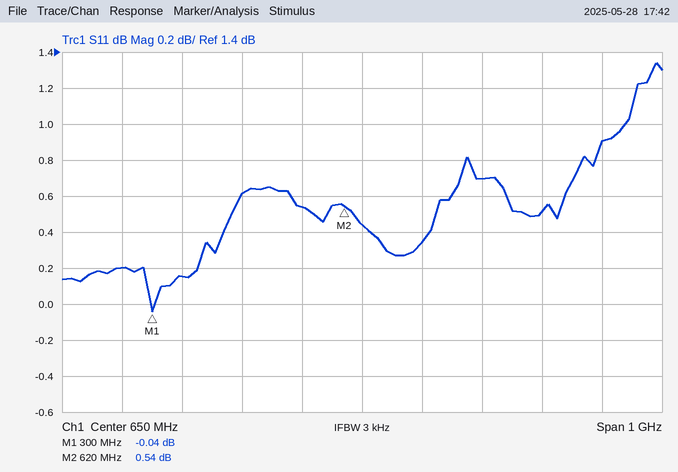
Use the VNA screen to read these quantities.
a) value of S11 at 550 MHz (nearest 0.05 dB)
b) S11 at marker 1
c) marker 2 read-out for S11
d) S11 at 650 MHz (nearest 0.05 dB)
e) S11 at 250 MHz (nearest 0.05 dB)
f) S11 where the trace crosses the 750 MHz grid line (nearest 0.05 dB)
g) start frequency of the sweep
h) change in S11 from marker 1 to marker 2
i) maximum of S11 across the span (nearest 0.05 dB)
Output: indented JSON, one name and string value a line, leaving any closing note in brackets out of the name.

{
  "value of S11 at 550 MHz": "0.55 dB",
  "S11 at marker 1": "-0.04 dB",
  "marker 2 read-out for S11": "0.54 dB",
  "S11 at 650 MHz": "0.45 dB",
  "S11 at 250 MHz": "0.20 dB",
  "S11 where the trace crosses the 750 MHz grid line": "0.35 dB",
  "start frequency of the sweep": "150 MHz",
  "change in S11 from marker 1 to marker 2": "0.58 dB",
  "maximum of S11 across the span": "1.35 dB"
}
